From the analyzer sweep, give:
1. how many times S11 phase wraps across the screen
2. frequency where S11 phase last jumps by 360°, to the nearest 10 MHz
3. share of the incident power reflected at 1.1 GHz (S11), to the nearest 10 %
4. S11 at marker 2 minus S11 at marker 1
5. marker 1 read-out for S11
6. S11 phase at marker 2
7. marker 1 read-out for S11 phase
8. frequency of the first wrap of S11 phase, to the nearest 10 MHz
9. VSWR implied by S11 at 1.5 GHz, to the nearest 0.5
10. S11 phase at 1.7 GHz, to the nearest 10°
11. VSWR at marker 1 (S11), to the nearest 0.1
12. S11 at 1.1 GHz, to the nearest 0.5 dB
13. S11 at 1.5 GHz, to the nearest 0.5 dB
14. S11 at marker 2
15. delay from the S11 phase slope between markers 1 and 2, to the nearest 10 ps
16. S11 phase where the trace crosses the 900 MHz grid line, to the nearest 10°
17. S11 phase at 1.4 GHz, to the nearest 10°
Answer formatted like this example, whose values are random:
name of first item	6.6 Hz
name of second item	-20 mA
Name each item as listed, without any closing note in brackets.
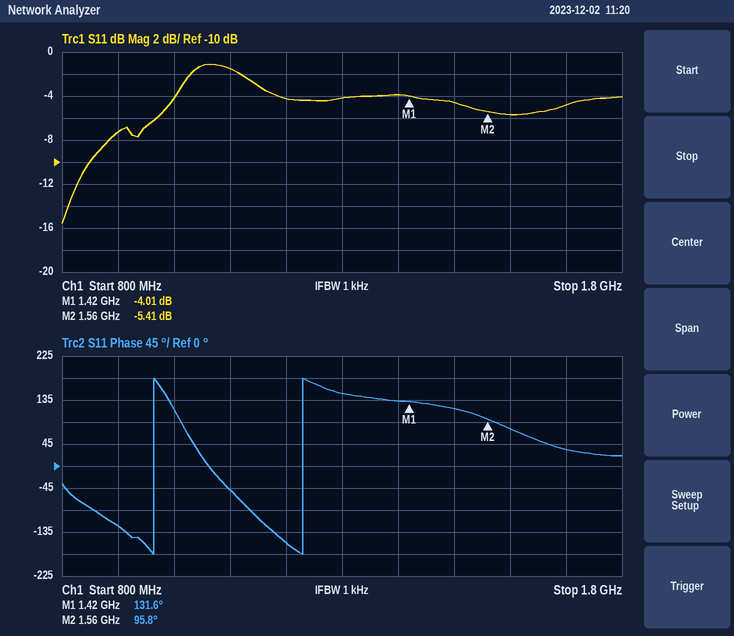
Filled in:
how many times S11 phase wraps across the screen	2
frequency where S11 phase last jumps by 360°, to the nearest 10 MHz	1.23 GHz
share of the incident power reflected at 1.1 GHz (S11), to the nearest 10 %	70 %
S11 at marker 2 minus S11 at marker 1	-1.40 dB
marker 1 read-out for S11	-4.01 dB
S11 phase at marker 2	95.8°
marker 1 read-out for S11 phase	131.6°
frequency of the first wrap of S11 phase, to the nearest 10 MHz	960 MHz
VSWR implied by S11 at 1.5 GHz, to the nearest 0.5	4.0
S11 phase at 1.7 GHz, to the nearest 10°	30°
VSWR at marker 1 (S11), to the nearest 0.1	4.4
S11 at 1.1 GHz, to the nearest 0.5 dB	-1.5 dB
S11 at 1.5 GHz, to the nearest 0.5 dB	-4.5 dB
S11 at marker 2	-5.41 dB
delay from the S11 phase slope between markers 1 and 2, to the nearest 10 ps	710 ps
S11 phase where the trace crosses the 900 MHz grid line, to the nearest 10°	-120°
S11 phase at 1.4 GHz, to the nearest 10°	130°
